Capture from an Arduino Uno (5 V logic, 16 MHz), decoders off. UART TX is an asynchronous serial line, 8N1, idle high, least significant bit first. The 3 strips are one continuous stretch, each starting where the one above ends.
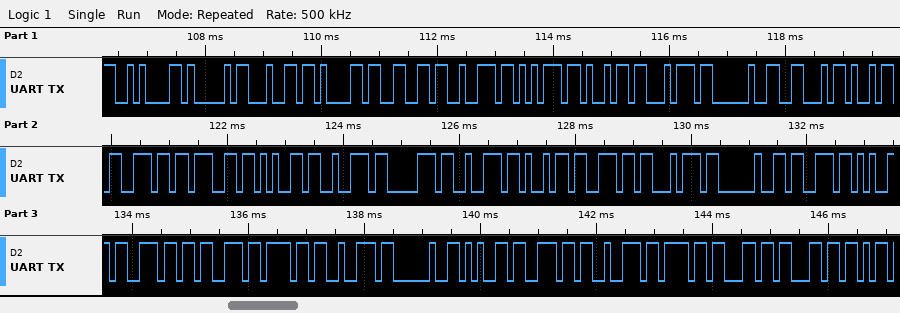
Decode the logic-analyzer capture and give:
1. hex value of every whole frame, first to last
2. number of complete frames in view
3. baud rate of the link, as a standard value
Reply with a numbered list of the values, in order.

1. 0A 41 64 61 66 72 75 69 74 20 46 69 6E 67 65 72 70 72 69 6E 74 20 73 65 6E 73 6F 72 20 65 6E 72 6F 6C 6C
2. 35
3. 9600 baud
